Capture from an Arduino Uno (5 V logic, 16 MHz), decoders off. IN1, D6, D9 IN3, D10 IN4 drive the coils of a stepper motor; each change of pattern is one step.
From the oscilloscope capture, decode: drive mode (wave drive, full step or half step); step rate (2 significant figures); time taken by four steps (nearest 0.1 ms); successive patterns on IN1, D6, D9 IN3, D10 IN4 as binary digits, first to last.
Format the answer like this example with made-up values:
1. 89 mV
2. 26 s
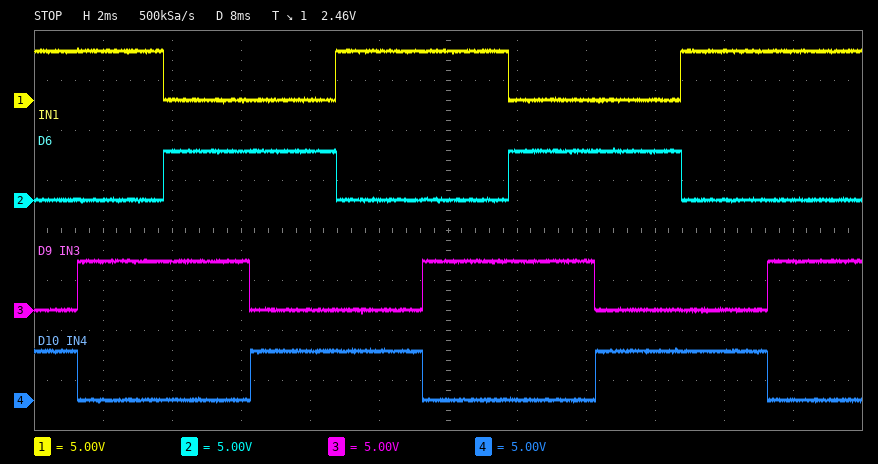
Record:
1. full step
2. 400 steps/s
3. 10.0 ms
4. 1001 1010 0110 0101 1001 1010 0110 0101 1001 1010
